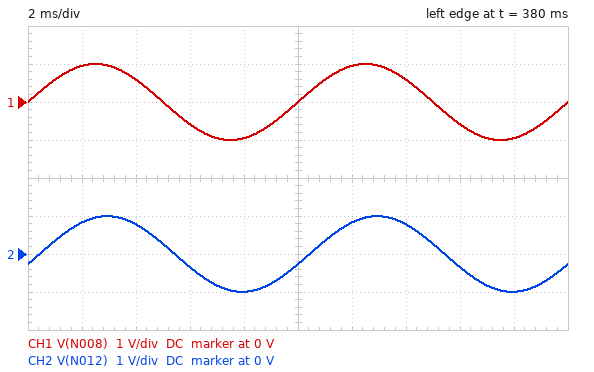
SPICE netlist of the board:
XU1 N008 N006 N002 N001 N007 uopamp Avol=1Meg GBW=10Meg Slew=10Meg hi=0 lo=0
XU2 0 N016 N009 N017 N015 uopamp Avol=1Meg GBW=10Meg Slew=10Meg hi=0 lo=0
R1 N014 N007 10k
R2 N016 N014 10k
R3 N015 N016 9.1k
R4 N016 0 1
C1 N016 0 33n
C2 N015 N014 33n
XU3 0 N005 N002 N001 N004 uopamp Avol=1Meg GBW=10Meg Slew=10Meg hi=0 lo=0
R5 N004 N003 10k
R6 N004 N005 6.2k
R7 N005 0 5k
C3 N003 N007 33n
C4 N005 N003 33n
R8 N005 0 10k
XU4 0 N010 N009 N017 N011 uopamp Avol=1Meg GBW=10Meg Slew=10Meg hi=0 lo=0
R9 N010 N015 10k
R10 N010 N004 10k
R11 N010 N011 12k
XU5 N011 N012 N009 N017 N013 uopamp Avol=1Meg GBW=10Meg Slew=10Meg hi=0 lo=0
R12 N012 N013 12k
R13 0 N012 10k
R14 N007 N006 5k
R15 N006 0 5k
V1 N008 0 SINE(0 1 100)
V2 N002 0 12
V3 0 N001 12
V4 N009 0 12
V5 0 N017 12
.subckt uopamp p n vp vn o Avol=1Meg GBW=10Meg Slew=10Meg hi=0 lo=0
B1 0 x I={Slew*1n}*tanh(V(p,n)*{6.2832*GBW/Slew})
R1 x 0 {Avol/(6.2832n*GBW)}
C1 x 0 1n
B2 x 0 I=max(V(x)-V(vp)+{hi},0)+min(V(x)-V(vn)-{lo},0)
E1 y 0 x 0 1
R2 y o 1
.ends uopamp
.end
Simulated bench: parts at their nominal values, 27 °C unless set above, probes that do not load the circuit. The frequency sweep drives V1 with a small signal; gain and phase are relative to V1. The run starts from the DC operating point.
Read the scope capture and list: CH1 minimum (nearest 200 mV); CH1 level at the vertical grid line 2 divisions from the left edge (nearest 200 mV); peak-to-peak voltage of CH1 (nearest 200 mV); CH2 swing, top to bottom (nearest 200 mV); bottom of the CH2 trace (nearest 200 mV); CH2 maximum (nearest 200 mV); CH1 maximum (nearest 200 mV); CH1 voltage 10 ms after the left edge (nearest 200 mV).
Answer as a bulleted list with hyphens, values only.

- -1.0 V
- 600 mV
- 2.0 V
- 2.0 V
- -1.0 V
- 1.0 V
- 1.0 V
- 0 V
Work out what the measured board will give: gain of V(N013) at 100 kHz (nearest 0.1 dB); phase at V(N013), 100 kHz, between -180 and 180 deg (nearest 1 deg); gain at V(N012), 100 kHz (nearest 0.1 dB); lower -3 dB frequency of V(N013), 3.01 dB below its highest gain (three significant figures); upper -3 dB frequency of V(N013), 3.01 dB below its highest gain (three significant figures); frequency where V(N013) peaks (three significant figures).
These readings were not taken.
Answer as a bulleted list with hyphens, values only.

- 54.1 dB
- 83 deg
- 47.3 dB
- 140 kHz
- 145 kHz
- 143 kHz
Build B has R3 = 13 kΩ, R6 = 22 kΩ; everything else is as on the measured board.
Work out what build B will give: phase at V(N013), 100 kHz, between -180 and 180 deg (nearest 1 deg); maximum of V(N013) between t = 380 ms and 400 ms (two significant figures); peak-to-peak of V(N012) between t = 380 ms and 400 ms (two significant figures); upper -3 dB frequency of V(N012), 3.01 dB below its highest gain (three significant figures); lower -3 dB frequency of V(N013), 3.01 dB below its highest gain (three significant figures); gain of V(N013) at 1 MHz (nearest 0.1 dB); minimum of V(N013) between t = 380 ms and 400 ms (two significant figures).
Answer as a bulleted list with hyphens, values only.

- -69 deg
- 2.9 V
- 2.6 V
- 97.8 kHz
- 94.1 kHz
- 33.7 dB
- -2.9 V
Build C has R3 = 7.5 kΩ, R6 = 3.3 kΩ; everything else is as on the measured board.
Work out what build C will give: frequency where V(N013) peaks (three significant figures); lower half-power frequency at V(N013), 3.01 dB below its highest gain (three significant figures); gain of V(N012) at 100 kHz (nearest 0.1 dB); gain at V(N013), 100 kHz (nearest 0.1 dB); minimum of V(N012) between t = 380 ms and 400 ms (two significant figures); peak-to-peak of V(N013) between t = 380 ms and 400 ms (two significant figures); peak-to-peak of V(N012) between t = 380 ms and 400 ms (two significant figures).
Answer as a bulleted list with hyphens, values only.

- 184 kHz
- 181 kHz
- 40.0 dB
- 46.8 dB
- -840 mV
- 3.7 V
- 1.7 V
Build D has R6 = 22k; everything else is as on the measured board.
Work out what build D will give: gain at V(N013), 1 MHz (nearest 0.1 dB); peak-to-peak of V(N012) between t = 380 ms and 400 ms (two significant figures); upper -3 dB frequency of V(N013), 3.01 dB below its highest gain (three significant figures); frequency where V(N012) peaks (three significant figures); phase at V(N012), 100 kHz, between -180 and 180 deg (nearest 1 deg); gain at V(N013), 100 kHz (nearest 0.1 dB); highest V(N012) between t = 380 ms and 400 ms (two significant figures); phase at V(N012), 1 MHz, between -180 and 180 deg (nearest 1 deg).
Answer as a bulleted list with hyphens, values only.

- 33.7 dB
- 1.8 V
- 97.8 kHz
- 95.9 kHz
- -69 deg
- 75.6 dB
- 900 mV
- -132 deg
